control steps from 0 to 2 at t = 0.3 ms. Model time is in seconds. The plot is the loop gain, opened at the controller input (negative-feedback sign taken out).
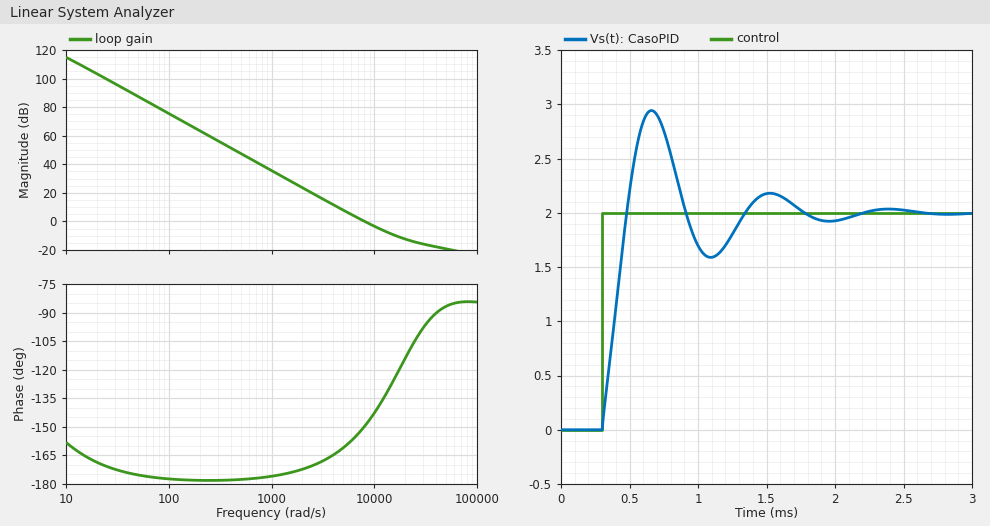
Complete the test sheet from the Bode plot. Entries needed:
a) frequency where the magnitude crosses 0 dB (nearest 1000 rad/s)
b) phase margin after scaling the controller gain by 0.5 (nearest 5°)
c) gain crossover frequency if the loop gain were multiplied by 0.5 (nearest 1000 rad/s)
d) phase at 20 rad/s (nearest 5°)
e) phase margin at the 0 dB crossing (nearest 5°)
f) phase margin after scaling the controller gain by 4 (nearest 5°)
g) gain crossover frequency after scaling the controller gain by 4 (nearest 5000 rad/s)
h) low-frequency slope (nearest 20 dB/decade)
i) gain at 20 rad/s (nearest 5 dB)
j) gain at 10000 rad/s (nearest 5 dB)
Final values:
8000 rad/s
20°
6000 rad/s
-170°
30°
65°
20000 rad/s
-40 dB/decade
105 dB
-5 dB
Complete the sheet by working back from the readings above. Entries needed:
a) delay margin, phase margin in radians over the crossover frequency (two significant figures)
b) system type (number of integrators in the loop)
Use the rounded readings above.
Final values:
0.000065 s
2
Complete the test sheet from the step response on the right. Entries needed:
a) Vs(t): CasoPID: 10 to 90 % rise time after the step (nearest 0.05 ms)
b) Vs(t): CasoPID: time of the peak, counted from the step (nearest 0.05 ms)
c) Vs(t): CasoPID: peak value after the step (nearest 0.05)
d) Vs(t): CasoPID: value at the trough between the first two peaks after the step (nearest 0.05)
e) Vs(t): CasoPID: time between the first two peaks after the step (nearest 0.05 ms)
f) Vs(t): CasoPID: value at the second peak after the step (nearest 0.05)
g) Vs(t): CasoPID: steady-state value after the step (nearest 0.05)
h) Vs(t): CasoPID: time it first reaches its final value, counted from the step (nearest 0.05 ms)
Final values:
0.15 ms
0.35 ms
2.95
1.60
0.85 ms
2.20
2.00
0.20 ms
